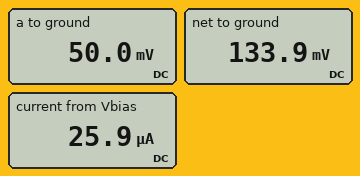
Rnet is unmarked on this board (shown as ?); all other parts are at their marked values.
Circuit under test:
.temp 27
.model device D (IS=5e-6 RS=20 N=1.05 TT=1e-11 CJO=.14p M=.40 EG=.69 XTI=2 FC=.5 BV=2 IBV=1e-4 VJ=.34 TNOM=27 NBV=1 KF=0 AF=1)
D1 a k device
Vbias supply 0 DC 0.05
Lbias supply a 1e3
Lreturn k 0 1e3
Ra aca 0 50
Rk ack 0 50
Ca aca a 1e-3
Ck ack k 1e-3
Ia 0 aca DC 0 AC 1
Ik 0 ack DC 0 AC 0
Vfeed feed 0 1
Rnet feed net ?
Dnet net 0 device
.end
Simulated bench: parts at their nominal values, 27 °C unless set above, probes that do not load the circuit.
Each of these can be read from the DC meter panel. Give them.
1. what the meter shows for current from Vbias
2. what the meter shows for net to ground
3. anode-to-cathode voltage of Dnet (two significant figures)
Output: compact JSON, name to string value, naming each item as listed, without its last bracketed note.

{"what the meter shows for current from Vbias": "25.9 µA", "what the meter shows for net to ground": "133.9 mV", "anode-to-cathode voltage of Dnet": "130 mV"}
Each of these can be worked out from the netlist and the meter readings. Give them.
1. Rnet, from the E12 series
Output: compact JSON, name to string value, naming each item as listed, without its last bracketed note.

{"Rnet, from the E12 series": "1.8 kΩ"}
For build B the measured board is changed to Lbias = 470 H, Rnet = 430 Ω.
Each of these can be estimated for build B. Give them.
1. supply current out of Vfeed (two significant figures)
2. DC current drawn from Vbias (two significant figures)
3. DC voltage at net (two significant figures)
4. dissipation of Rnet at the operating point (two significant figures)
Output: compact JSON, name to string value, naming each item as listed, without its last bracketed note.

{"supply current out of Vfeed": "1.9 mA", "DC current drawn from Vbias": "26 µA", "DC voltage at net": "200 mV", "dissipation of Rnet at the operating point": "1.5 mW"}
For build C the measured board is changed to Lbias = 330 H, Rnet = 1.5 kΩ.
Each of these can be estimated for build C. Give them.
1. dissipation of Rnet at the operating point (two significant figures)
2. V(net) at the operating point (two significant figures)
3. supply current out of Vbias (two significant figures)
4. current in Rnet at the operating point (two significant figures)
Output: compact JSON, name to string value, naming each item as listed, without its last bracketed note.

{"dissipation of Rnet at the operating point": "490 µW", "V(net) at the operating point": "140 mV", "supply current out of Vbias": "26 µA", "current in Rnet at the operating point": "570 µA"}
